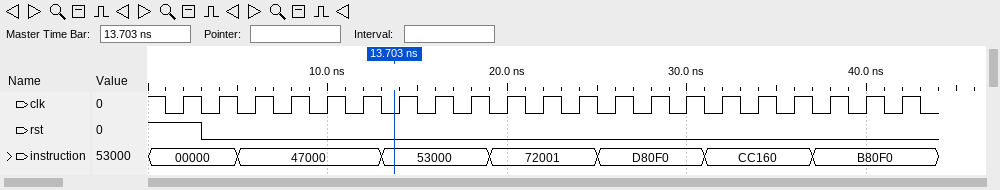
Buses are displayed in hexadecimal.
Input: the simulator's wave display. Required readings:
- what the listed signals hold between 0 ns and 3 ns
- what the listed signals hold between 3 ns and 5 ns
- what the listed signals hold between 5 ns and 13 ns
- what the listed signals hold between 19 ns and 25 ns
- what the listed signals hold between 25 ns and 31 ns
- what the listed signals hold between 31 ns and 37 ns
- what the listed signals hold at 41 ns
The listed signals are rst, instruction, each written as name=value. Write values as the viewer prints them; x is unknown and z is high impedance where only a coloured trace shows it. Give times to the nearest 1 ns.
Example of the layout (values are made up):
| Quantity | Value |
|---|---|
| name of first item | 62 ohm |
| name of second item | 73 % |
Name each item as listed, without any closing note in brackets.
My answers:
| Quantity | Value |
|---|---|
| what the listed signals hold between 0 ns and 3 ns | rst=1, instruction=00000 |
| what the listed signals hold between 3 ns and 5 ns | rst=0, instruction=00000 |
| what the listed signals hold between 5 ns and 13 ns | rst=0, instruction=47000 |
| what the listed signals hold between 19 ns and 25 ns | rst=0, instruction=72001 |
| what the listed signals hold between 25 ns and 31 ns | rst=0, instruction=D80F0 |
| what the listed signals hold between 31 ns and 37 ns | rst=0, instruction=CC160 |
| what the listed signals hold at 41 ns | rst=0, instruction=B80F0 |
